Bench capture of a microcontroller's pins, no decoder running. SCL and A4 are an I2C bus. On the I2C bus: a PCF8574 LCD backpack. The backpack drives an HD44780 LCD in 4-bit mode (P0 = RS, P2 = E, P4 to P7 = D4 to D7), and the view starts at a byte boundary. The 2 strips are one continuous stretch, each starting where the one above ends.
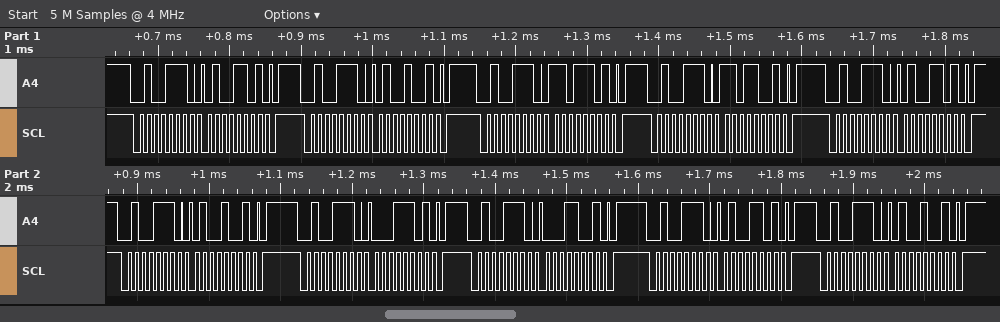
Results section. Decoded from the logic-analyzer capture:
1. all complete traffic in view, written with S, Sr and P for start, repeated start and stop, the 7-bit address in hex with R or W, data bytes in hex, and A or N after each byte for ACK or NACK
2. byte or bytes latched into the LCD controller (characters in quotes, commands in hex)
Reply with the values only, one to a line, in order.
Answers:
S 27W A 4D A P S 27W A 49 A P S 27W A DD A P S 27W A D9 A P S 27W A 4D A P S 27W A 49 A P S 27W A 1D A P S 27W A 19 A P S 27W A 4D A P S 27W A 49 A P
'M' 'A'
